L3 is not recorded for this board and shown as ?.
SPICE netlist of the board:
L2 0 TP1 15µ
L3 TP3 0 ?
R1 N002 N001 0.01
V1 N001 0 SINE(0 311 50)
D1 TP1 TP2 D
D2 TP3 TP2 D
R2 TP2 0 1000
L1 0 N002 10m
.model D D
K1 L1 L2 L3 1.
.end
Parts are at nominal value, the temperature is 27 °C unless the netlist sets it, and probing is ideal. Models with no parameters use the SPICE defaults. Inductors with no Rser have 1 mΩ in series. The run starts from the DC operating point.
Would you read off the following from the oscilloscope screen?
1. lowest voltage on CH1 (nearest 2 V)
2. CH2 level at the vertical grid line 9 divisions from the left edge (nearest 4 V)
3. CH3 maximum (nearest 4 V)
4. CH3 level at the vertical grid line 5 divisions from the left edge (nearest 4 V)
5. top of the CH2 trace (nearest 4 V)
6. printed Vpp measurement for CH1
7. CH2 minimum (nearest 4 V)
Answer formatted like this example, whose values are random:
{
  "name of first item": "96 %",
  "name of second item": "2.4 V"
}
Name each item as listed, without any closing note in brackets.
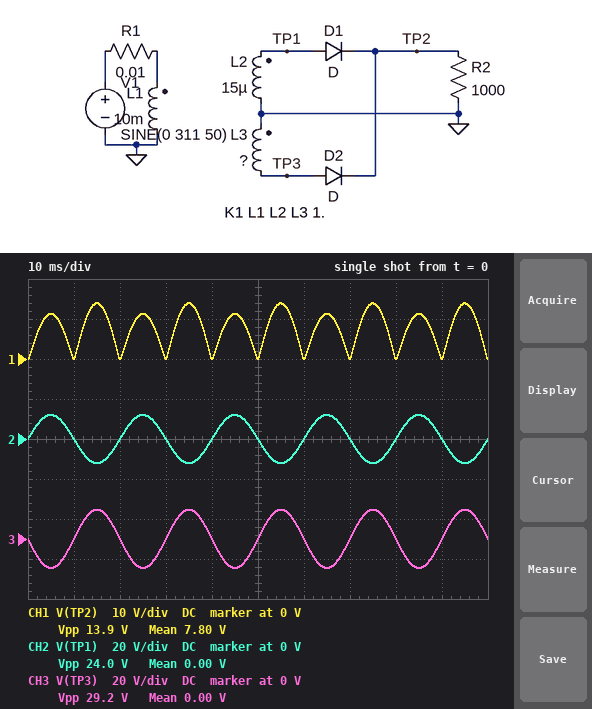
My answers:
{
  "lowest voltage on CH1": "0 V",
  "CH2 level at the vertical grid line 9 divisions from the left edge": "0 V",
  "CH3 maximum": "16 V",
  "CH3 level at the vertical grid line 5 divisions from the left edge": "0 V",
  "top of the CH2 trace": "12 V",
  "printed Vpp measurement for CH1": "13.9 V",
  "CH2 minimum": "-12 V"
}
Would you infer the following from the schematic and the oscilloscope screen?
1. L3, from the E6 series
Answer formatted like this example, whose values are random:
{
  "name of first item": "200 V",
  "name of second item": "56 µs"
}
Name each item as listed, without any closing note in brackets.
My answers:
{
  "L3, from the E6 series": "22 µH"
}
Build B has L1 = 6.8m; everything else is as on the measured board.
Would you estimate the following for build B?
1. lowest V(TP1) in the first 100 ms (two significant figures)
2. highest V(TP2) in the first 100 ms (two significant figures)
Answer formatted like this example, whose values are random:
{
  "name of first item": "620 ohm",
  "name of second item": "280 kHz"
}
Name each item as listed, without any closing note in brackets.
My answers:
{
  "lowest V(TP1) in the first 100 ms": "-15 V",
  "highest V(TP2) in the first 100 ms": "17 V"
}
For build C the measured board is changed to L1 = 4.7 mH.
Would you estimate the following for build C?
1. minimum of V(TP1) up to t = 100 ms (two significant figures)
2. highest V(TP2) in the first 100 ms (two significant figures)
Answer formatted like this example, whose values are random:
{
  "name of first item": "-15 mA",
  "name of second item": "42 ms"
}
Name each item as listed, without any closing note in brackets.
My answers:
{
  "minimum of V(TP1) up to t = 100 ms": "-18 V",
  "highest V(TP2) in the first 100 ms": "21 V"
}
